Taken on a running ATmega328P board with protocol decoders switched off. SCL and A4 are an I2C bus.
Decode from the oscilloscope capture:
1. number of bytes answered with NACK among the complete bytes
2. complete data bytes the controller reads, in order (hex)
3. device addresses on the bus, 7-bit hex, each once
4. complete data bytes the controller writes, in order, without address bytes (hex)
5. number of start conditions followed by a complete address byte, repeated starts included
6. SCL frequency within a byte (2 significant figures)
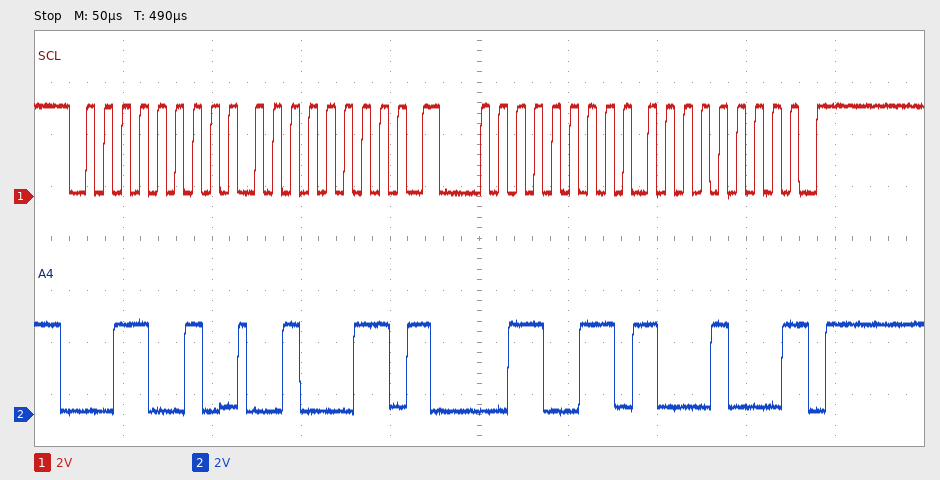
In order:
1
88
0x19
23
2
100 kHz
